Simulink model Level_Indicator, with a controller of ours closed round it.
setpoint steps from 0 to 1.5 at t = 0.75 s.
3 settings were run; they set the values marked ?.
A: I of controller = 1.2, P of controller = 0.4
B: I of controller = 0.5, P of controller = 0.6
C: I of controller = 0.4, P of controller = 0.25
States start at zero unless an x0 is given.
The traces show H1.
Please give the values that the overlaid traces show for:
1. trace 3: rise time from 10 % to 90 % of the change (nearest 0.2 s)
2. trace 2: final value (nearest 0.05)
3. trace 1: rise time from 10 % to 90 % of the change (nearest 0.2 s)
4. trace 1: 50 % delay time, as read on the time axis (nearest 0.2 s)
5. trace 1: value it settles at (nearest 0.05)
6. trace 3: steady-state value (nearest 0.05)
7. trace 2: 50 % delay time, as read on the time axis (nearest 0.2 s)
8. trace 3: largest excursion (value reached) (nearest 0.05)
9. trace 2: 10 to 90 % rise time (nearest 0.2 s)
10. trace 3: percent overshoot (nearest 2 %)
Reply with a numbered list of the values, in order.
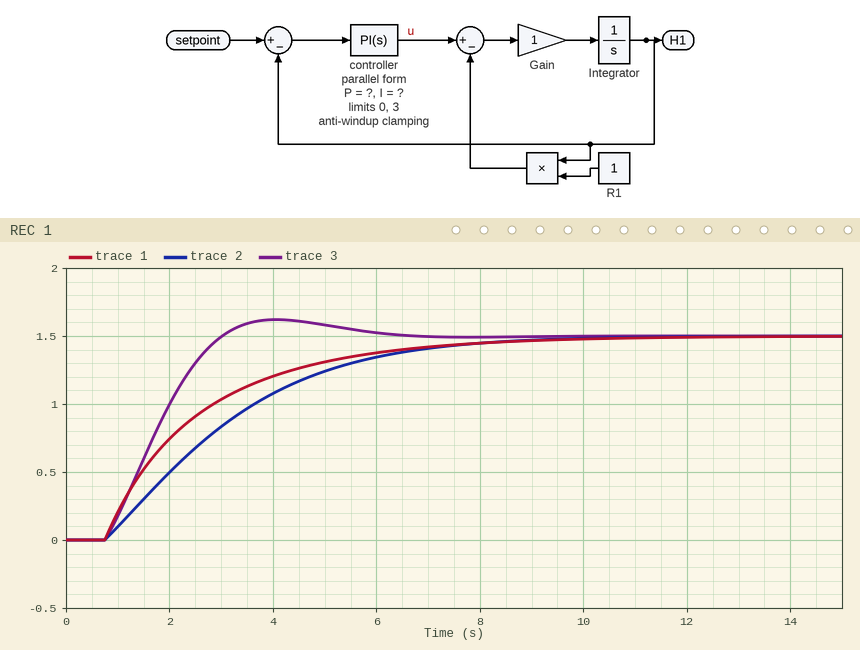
1. 1.6 s
2. 1.50
3. 4.6 s
4. 2.0 s
5. 1.50
6. 1.50
7. 2.8 s
8. 1.60
9. 5.0 s
10. 8 %
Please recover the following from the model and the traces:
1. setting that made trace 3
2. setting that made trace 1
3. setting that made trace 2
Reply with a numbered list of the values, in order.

1. A
2. B
3. C
